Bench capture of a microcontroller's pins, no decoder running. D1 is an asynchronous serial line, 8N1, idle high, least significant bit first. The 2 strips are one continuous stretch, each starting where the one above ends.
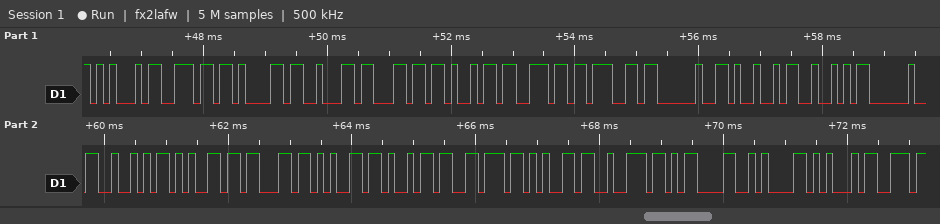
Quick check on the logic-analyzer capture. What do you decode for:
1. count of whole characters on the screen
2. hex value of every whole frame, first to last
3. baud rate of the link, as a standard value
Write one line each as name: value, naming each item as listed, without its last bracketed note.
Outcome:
count of whole characters on the screen: 23
hex value of every whole frame, first to last: 0x45 0x6E 0x61 0x62 0x6C 0x69 0x6E 0x67 0x20 0x49 0x52 0x20 0x52 0x65 0x63 0x65 0x69 0x76 0x65 0x72 0x0D 0x0A 0x45
baud rate of the link, as a standard value: 9600 baud
